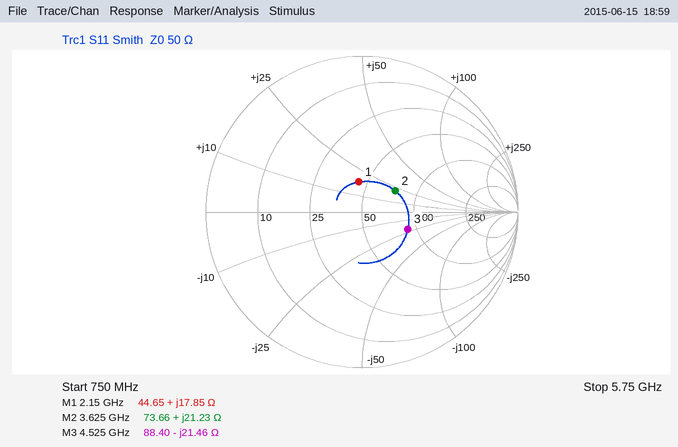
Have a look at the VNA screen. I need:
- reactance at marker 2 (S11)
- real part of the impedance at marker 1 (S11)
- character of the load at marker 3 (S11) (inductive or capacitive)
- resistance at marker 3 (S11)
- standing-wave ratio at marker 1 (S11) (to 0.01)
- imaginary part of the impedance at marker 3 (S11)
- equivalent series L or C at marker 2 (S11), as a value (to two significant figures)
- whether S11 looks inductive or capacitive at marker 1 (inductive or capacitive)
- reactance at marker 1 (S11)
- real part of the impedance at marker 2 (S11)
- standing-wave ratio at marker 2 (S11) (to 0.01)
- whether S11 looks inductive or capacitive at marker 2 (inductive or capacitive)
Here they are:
+21.23 Ω
44.65 Ω
capacitive
88.40 Ω
1.48
-21.46 Ω
930 pH
inductive
+17.85 Ω
73.66 Ω
1.68
inductive
